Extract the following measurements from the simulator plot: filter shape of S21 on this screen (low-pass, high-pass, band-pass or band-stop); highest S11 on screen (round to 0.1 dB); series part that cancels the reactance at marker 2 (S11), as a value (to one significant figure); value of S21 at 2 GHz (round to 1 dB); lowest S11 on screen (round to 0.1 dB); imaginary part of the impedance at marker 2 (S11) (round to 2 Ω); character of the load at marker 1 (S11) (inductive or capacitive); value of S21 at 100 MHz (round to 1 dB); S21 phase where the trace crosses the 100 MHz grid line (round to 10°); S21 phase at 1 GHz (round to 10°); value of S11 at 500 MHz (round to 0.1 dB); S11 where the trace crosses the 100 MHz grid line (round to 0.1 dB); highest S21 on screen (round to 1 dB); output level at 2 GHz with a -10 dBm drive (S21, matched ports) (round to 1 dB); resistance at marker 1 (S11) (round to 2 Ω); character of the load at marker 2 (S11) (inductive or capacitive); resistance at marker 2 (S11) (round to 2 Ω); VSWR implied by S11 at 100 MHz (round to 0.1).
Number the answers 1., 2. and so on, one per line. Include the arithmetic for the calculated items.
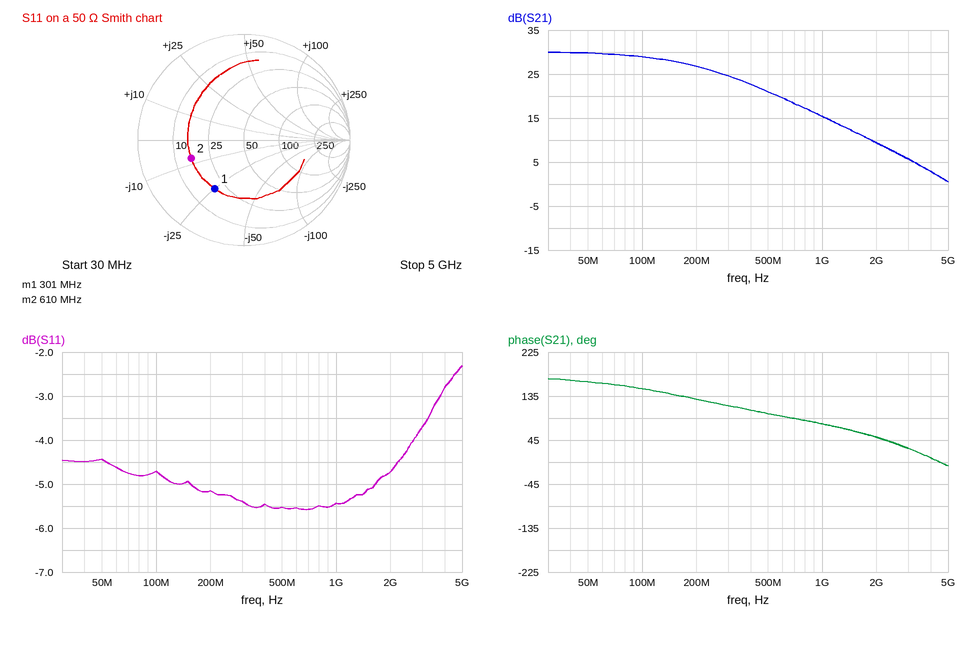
1. low-pass
2. -2.3 dB
3. L = 8 Ω/(2π × 610 MHz) ≈ 2 nH
4. 9 dB
5. -5.6 dB
6. -8 Ω
7. capacitive
8. 29 dB
9. 150°
10. 80°
11. -5.5 dB
12. -4.7 dB
13. 30 dB
14. -10 dBm + (9 dB) = -1 dBm
15. 20 Ω
16. capacitive
17. 16 Ω
18. |Γ| = 10^(-4.7/20) = 0.5821; VSWR = (1 + 0.5821)/(1 − 0.5821) ≈ 3.8
